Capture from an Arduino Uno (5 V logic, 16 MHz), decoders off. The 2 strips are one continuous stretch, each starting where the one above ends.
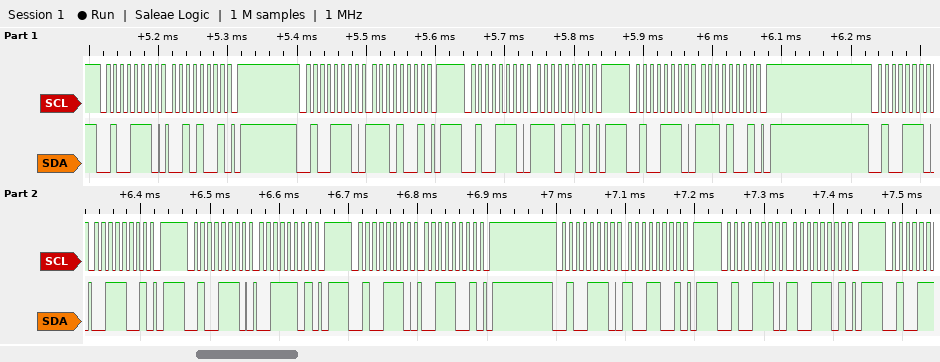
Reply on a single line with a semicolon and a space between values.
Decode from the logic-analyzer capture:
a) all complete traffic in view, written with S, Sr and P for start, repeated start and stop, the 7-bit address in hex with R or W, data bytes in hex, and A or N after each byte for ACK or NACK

S 27W A 29 A P S 27W A E9 A P S 27W A ED A P S 27W A E9 A P S 27W A 39 A P S 27W A 3D A P S 27W A 39 A P S 27W A 99 A P S 27W A 9D A P
